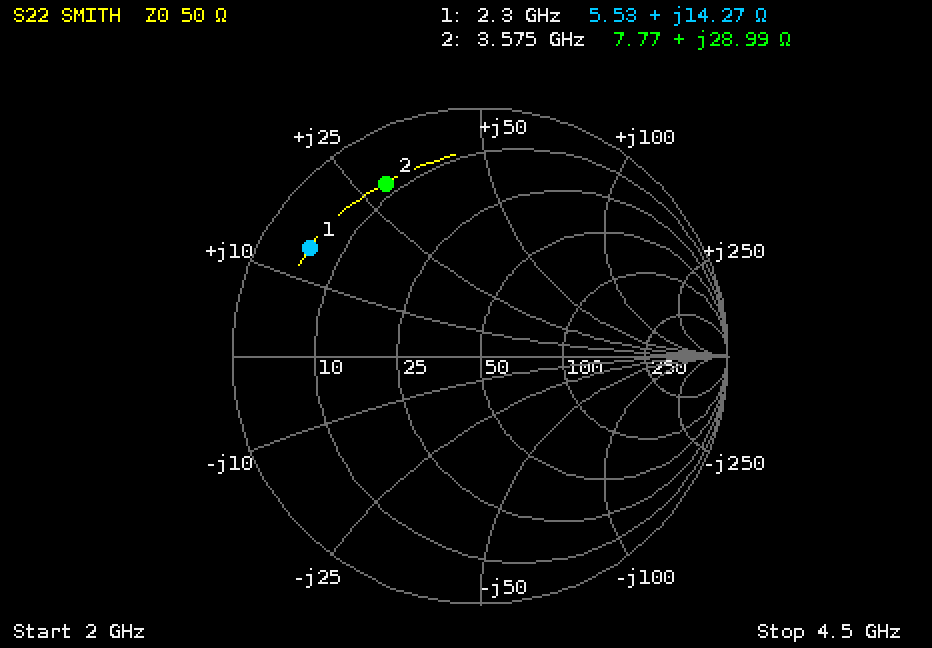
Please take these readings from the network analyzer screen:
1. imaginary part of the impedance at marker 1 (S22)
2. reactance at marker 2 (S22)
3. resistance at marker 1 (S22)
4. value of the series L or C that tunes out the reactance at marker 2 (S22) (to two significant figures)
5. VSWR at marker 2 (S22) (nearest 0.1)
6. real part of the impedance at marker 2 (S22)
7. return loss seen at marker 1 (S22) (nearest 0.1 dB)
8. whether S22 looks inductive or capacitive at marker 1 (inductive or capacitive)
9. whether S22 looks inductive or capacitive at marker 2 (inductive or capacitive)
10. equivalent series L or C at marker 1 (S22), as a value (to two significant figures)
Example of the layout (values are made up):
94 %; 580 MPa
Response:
+14.27 Ω; +28.99 Ω; 5.53 Ω; 1.5 pF; 8.6; 7.77 Ω; 1.8 dB; inductive; inductive; 990 pH
